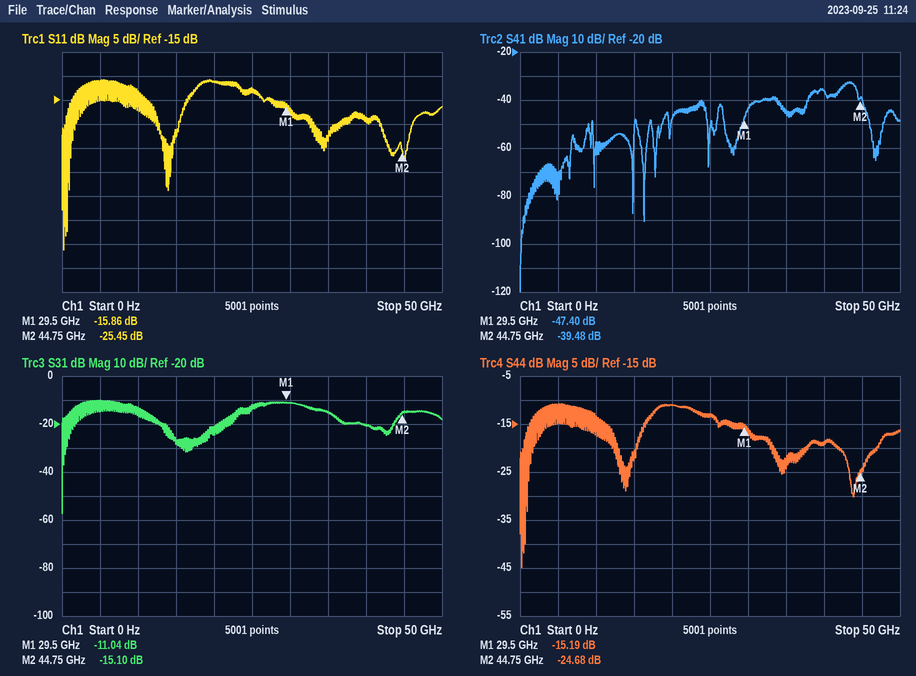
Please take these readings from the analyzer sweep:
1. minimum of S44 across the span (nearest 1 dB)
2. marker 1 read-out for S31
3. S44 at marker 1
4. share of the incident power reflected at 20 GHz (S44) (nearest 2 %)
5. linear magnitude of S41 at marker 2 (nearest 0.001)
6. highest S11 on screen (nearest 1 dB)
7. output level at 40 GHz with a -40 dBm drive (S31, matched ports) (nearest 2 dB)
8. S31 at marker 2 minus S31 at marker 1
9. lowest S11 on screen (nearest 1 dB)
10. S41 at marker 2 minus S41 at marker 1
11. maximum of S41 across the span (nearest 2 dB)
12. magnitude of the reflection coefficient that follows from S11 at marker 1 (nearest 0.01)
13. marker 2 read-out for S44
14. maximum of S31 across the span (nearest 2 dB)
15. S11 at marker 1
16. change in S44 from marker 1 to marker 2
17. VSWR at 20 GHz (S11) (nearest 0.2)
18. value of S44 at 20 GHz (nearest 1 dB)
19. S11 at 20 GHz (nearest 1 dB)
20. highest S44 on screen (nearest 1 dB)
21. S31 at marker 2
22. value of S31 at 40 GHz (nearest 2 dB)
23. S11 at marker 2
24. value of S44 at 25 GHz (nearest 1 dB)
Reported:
-45 dB
-11.04 dB
-15.19 dB
8 %
0.011
-11 dB
-60 dBm
-4.06 dB
-46 dB
7.92 dB
-32 dB
0.16
-24.68 dB
-10 dB
-15.86 dB
-9.49 dB
1.8
-11 dB
-11 dB
-11 dB
-15.10 dB
-20 dB
-25.45 dB
-13 dB
